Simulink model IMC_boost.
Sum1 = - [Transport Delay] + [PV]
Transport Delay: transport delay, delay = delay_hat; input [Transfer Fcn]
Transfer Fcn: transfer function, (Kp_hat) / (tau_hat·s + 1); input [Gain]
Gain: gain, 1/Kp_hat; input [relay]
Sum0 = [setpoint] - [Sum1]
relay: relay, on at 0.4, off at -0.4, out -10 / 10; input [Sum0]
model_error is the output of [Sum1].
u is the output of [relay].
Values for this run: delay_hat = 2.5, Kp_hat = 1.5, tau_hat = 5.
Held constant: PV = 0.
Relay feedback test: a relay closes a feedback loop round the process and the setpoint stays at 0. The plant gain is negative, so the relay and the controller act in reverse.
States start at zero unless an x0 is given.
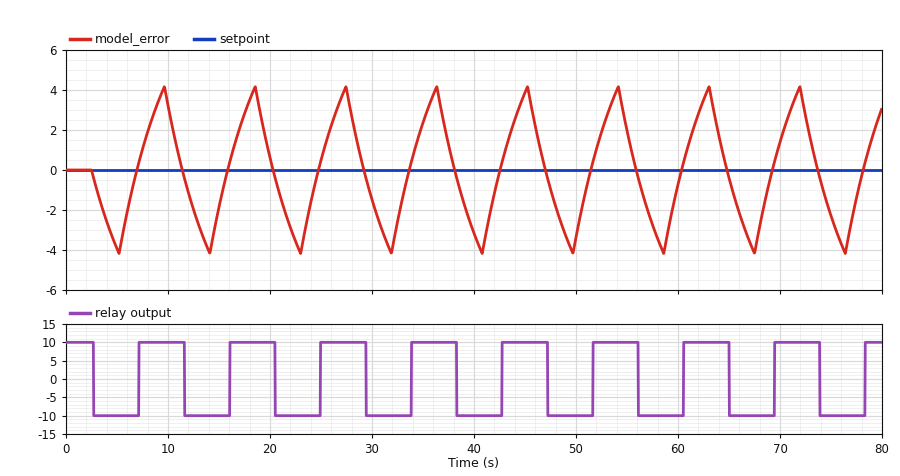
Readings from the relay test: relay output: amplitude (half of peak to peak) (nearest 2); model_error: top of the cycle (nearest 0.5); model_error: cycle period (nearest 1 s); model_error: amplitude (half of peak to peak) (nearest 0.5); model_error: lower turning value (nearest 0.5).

10
4.0
9 s
4.0
-4.0
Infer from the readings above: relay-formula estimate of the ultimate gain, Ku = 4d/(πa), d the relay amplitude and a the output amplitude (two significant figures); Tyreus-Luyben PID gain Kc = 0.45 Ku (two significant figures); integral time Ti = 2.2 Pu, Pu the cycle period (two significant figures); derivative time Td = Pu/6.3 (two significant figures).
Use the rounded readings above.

3.2
1.4
20 s
1.4 s
